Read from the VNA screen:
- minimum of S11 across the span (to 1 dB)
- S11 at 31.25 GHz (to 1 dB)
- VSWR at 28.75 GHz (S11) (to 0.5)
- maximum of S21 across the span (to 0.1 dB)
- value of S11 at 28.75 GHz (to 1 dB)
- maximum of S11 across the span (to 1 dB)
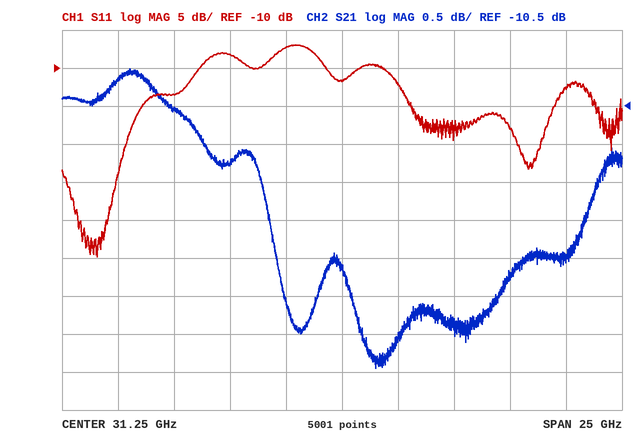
-35 dB
-12 dB
2.5
-10.0 dB
-7 dB
-7 dB
